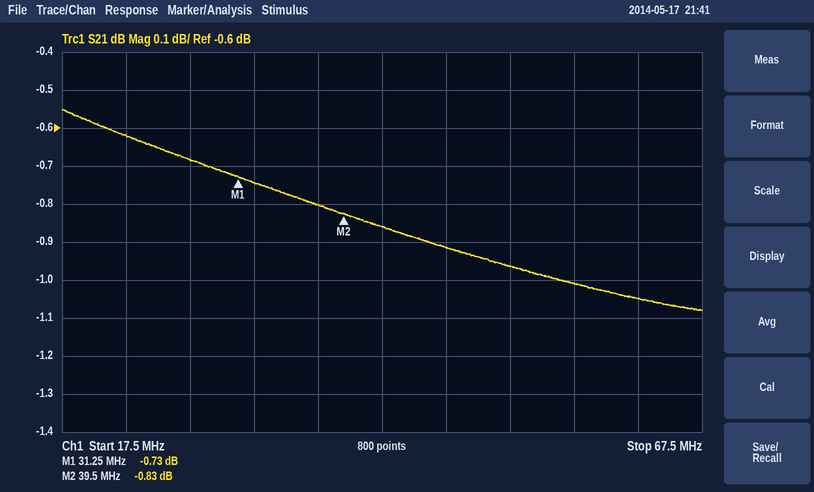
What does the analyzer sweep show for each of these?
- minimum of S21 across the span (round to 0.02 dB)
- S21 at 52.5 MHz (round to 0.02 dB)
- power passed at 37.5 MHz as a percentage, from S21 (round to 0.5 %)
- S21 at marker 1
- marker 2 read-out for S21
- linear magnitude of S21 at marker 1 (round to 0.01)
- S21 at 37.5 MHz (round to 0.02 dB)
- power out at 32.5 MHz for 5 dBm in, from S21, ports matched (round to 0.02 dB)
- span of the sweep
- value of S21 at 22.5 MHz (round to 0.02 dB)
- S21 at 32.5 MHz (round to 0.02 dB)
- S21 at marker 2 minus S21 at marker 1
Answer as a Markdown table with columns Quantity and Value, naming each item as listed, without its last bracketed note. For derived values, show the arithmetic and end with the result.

| Quantity | Value |
|---|---|
| minimum of S21 across the span | -1.08 dB |
| S21 at 52.5 MHz | -0.96 dB |
| power passed at 37.5 MHz as a percentage, from S21 | 10^(-0.8/10) ≈ 83.2 %, so 83.0 % to the nearest 0.5 % |
| S21 at marker 1 | -0.73 dB |
| marker 2 read-out for S21 | -0.83 dB |
| linear magnitude of S21 at marker 1 | 10^(-0.73/20) ≈ 0.92 |
| S21 at 37.5 MHz | -0.80 dB |
| power out at 32.5 MHz for 5 dBm in, from S21, ports matched | 5 dBm + (-0.74 dB) = 4.26 dBm |
| span of the sweep | 50 MHz |
| value of S21 at 22.5 MHz | -0.62 dB |
| S21 at 32.5 MHz | -0.74 dB |
| S21 at marker 2 minus S21 at marker 1 | -0.83 − (-0.73) = -0.10 dB |
